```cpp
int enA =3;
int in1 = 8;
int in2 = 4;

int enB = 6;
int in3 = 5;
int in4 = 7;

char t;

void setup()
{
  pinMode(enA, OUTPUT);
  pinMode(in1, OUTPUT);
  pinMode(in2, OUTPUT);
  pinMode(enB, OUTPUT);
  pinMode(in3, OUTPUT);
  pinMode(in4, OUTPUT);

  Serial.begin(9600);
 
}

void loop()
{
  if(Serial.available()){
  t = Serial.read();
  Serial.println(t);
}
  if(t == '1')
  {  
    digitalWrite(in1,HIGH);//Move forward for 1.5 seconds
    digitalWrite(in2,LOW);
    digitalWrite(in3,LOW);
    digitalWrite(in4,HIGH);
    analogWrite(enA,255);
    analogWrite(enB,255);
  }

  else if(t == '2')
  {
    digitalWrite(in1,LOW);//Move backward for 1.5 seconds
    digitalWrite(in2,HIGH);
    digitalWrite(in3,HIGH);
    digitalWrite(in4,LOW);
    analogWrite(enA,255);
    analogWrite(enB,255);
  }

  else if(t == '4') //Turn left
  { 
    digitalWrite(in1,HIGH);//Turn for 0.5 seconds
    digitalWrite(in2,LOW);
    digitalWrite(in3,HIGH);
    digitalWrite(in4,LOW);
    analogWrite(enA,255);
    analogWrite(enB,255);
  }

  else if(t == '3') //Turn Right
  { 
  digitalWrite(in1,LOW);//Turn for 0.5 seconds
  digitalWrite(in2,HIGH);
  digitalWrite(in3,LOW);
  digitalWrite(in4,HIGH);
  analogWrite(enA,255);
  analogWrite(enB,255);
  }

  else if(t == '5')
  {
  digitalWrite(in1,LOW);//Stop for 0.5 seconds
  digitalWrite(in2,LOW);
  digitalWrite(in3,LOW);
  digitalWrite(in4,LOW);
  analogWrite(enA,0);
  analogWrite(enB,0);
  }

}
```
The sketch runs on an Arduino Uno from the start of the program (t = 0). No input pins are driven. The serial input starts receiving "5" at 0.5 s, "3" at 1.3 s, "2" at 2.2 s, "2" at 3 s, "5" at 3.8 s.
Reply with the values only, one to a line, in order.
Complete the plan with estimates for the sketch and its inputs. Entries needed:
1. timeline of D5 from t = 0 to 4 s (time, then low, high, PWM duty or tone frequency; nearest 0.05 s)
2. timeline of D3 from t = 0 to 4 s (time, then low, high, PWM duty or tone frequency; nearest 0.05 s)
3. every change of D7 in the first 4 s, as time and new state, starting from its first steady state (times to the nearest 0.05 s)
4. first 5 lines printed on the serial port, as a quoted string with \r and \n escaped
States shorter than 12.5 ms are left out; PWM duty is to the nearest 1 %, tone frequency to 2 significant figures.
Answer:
0 s low; 2.2 s high; 3.8 s low
0 s low; 1.3 s high; 3.8 s low
0 s low; 1.3 s high; 2.2 s low
"5\r\n3\r\n2\r\n2\r\n5\r\n"
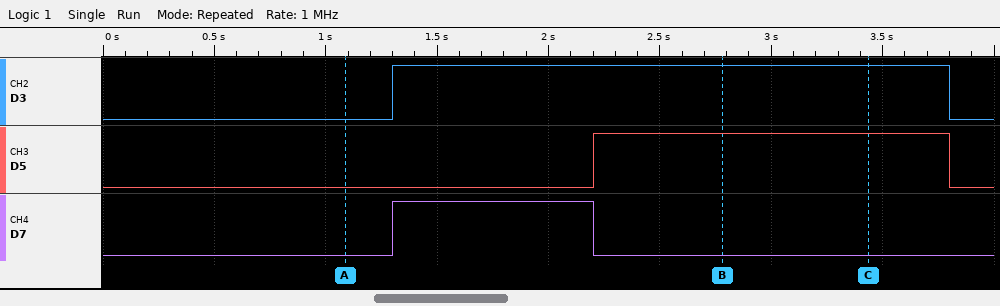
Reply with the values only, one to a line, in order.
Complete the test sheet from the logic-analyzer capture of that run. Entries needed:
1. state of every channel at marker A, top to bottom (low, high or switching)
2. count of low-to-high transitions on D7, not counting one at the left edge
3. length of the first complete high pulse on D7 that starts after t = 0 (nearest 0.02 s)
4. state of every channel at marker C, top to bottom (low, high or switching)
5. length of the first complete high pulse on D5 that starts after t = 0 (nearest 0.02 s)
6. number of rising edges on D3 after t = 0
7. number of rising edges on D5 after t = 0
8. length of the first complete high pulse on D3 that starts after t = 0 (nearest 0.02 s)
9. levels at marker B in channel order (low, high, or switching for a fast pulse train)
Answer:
D3 low, D5 low, D7 low
1
0.90 s
D3 high, D5 high, D7 low
1.60 s
1
1
2.50 s
D3 high, D5 high, D7 low
